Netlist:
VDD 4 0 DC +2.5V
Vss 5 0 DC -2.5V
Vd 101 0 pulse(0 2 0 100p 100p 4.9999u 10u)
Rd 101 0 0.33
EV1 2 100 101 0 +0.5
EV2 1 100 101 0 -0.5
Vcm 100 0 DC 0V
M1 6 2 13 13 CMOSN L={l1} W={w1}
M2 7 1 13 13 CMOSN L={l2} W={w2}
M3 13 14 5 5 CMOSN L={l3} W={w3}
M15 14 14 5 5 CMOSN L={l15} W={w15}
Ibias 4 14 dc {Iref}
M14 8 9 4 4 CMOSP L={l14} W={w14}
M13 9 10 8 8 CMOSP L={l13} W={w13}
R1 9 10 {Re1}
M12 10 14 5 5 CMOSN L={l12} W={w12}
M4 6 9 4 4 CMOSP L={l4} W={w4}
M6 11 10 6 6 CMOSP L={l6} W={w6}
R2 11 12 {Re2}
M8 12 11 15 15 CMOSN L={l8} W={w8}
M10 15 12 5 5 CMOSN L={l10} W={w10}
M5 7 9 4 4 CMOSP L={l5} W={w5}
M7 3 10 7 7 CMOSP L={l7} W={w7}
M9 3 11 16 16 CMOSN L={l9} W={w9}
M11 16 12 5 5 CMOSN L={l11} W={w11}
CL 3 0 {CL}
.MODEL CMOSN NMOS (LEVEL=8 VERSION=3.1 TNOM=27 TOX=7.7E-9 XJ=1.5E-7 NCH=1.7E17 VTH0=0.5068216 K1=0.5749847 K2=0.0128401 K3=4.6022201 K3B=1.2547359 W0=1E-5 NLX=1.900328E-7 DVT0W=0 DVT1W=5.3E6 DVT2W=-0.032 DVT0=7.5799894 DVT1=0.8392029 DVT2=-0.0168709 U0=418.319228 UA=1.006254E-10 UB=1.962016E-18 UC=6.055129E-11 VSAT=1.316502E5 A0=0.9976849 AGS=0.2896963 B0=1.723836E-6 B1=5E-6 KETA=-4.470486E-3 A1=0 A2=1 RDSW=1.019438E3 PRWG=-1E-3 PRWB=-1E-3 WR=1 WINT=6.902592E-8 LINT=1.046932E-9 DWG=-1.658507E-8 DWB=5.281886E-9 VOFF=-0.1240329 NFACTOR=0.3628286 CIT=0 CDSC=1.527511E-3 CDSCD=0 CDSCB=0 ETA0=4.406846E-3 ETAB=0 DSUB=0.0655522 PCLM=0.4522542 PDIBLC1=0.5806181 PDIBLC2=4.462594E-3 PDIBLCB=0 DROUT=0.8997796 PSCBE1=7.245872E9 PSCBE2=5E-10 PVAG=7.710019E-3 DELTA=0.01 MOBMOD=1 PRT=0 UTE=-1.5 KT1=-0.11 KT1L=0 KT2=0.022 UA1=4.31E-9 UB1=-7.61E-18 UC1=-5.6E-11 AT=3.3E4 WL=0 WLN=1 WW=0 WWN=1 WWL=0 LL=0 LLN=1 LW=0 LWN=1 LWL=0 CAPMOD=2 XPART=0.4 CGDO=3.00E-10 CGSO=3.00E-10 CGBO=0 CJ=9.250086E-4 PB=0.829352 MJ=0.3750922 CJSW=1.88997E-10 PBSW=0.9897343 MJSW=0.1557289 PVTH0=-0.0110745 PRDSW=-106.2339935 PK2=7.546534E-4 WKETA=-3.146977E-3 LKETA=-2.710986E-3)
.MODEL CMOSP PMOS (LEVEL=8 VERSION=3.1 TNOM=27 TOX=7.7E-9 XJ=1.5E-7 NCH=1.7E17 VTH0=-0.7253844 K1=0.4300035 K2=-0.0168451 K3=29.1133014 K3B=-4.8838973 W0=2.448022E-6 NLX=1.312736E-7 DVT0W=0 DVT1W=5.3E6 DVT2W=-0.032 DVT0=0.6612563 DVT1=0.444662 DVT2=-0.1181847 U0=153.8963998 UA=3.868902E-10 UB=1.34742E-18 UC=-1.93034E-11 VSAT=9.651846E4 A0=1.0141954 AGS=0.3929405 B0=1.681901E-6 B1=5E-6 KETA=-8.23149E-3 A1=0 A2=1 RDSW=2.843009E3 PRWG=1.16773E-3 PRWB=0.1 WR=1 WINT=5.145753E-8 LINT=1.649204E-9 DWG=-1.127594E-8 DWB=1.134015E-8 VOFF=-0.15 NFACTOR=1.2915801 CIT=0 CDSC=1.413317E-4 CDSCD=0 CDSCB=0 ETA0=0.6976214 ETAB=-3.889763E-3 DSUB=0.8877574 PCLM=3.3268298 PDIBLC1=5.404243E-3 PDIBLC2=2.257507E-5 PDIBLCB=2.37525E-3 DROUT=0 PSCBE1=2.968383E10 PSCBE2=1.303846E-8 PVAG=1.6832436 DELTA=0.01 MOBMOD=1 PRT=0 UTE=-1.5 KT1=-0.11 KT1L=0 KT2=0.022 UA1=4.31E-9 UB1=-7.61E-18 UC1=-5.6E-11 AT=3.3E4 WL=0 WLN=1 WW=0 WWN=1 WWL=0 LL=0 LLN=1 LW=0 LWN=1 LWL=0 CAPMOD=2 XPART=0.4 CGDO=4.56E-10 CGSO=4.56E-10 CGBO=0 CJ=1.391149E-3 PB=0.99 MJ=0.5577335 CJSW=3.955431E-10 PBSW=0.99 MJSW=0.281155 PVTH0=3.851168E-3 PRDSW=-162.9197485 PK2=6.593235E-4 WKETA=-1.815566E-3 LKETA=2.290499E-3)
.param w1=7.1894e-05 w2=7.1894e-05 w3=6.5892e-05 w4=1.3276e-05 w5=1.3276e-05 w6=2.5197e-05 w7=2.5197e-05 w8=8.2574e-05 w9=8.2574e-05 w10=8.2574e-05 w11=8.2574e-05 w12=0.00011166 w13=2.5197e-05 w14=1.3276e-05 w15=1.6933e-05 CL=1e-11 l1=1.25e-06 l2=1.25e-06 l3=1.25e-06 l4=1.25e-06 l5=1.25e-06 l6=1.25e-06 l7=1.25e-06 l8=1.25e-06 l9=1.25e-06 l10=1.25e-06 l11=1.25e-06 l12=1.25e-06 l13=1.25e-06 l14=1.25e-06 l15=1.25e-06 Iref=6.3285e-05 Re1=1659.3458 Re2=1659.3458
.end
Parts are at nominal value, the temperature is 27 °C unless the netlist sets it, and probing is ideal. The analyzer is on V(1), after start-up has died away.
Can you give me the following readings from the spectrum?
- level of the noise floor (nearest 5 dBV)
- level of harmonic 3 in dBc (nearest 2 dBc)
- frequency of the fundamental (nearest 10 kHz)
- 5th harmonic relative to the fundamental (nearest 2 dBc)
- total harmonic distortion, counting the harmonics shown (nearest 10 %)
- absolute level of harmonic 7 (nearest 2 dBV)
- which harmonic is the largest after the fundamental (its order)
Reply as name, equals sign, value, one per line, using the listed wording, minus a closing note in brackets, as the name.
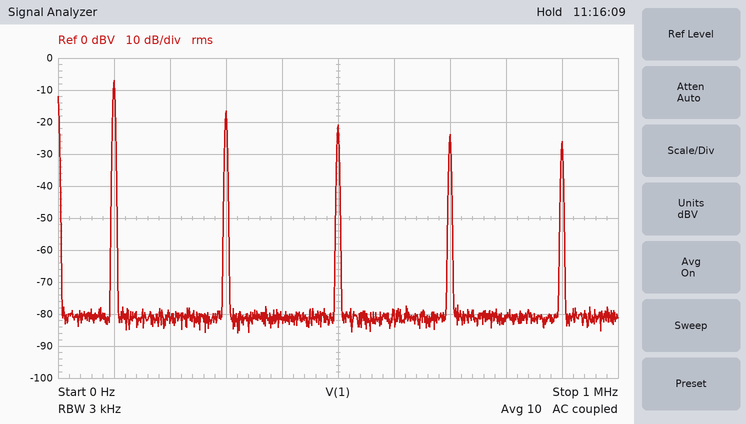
level of the noise floor = -80 dBV
level of harmonic 3 in dBc = -10 dBc
frequency of the fundamental = 100 kHz
5th harmonic relative to the fundamental = -14 dBc
total harmonic distortion, counting the harmonics shown = 40 %
absolute level of harmonic 7 = -24 dBV
which harmonic is the largest after the fundamental = 3
